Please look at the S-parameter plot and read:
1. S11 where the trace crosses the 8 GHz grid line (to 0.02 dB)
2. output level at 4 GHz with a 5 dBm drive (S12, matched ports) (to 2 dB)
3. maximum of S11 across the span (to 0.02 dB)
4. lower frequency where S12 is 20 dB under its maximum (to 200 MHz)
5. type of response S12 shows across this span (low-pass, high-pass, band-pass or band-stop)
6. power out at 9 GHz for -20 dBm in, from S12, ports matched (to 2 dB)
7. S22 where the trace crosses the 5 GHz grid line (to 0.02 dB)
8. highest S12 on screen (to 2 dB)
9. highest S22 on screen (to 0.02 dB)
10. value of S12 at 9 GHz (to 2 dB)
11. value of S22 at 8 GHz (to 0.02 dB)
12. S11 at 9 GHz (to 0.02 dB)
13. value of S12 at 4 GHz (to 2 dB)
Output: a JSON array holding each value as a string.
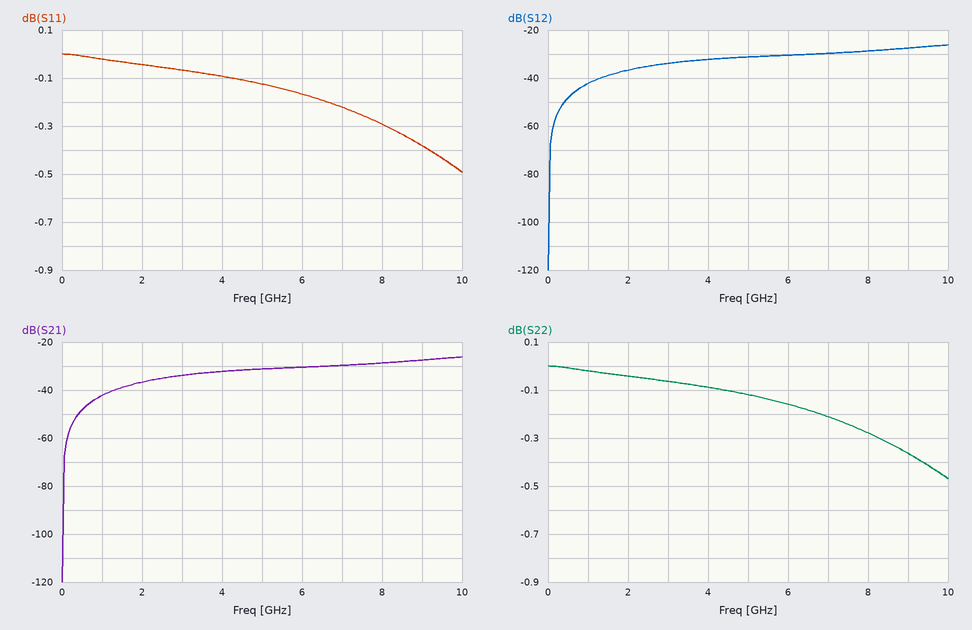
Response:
["-0.30 dB", "-28 dBm", "0.00 dB", "600 MHz", "high-pass", "-48 dBm", "-0.12 dB", "-26 dB", "0.00 dB", "-28 dB", "-0.28 dB", "-0.38 dB", "-32 dB"]
